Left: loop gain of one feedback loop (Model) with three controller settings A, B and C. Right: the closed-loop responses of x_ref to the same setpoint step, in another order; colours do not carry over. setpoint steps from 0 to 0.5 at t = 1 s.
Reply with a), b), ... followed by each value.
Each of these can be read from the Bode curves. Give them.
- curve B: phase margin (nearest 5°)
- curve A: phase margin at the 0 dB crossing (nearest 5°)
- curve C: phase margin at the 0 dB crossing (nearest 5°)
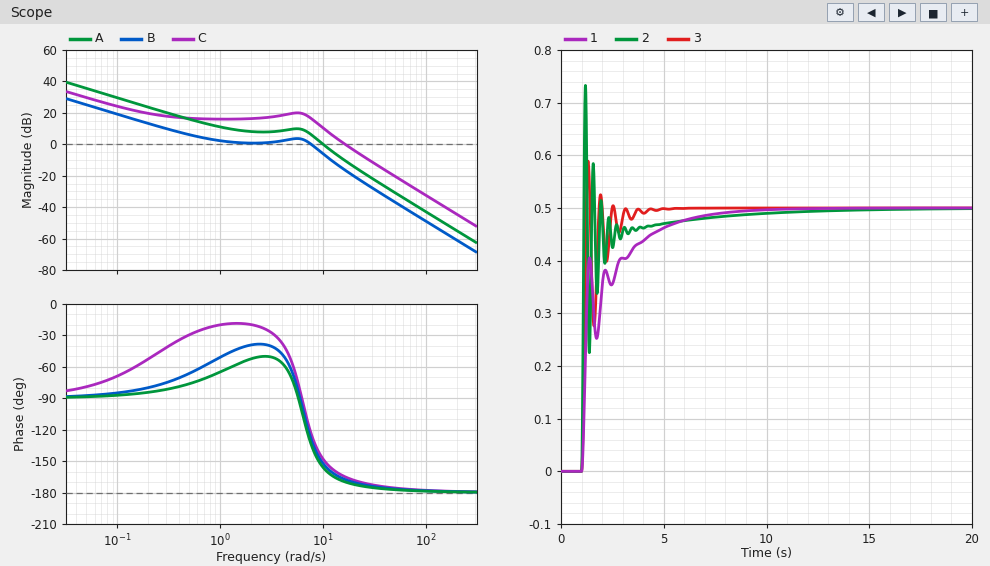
a) 50°
b) 25°
c) 15°
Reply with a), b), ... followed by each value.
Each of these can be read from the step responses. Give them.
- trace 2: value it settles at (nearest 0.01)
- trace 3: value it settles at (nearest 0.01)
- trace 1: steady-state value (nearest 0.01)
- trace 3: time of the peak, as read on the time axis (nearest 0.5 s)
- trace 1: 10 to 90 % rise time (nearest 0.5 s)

a) 0.50
b) 0.50
c) 0.50
d) 1.5 s
e) 3.5 s
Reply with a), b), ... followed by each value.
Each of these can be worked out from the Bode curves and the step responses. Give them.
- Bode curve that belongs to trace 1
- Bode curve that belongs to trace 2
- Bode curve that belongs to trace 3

a) B
b) C
c) A
